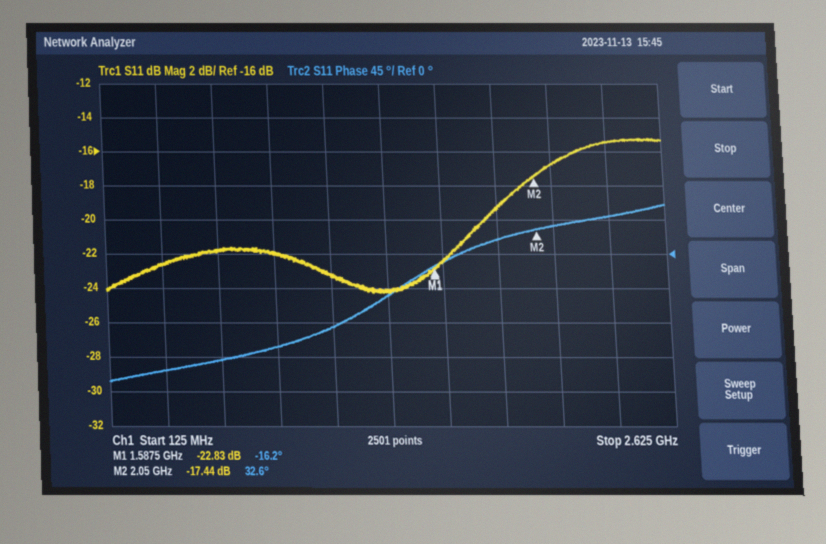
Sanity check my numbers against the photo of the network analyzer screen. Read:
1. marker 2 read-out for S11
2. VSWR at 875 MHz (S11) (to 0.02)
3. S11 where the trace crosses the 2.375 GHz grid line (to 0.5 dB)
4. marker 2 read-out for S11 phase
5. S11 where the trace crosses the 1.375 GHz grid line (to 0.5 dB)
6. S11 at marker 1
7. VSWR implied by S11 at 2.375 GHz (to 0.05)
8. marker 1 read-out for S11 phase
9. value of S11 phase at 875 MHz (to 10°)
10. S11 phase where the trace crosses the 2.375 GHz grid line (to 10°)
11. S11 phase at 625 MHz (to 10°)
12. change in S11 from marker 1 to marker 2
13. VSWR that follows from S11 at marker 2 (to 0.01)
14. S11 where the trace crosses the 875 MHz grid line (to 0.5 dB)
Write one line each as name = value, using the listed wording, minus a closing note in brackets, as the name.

marker 2 read-out for S11 = -17.44 dB
VSWR at 875 MHz (S11) = 1.18
S11 where the trace crosses the 2.375 GHz grid line = -15.5 dB
marker 2 read-out for S11 phase = 32.6°
S11 where the trace crosses the 1.375 GHz grid line = -24.0 dB
S11 at marker 1 = -22.83 dB
VSWR implied by S11 at 2.375 GHz = 1.40
marker 1 read-out for S11 phase = -16.2°
value of S11 phase at 875 MHz = -120°
S11 phase where the trace crosses the 2.375 GHz grid line = 50°
S11 phase at 625 MHz = -140°
change in S11 from marker 1 to marker 2 = 5.39 dB
VSWR that follows from S11 at marker 2 = 1.31
S11 where the trace crosses the 875 MHz grid line = -22.0 dB
